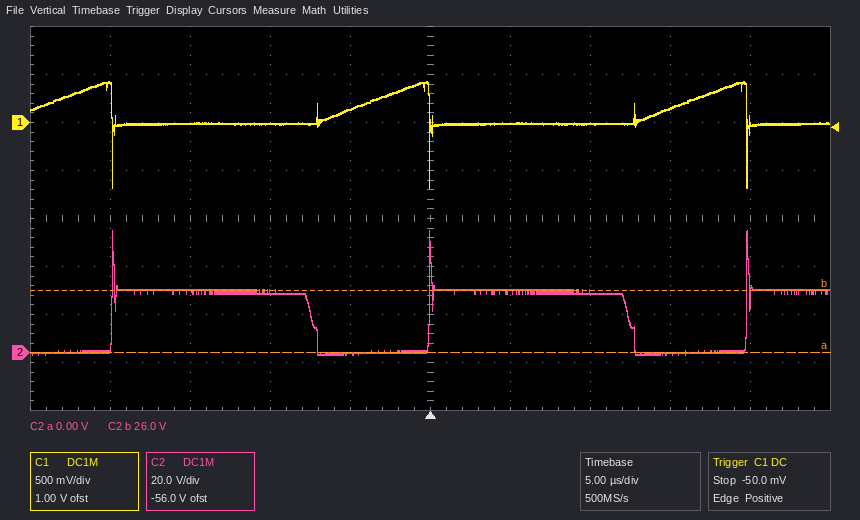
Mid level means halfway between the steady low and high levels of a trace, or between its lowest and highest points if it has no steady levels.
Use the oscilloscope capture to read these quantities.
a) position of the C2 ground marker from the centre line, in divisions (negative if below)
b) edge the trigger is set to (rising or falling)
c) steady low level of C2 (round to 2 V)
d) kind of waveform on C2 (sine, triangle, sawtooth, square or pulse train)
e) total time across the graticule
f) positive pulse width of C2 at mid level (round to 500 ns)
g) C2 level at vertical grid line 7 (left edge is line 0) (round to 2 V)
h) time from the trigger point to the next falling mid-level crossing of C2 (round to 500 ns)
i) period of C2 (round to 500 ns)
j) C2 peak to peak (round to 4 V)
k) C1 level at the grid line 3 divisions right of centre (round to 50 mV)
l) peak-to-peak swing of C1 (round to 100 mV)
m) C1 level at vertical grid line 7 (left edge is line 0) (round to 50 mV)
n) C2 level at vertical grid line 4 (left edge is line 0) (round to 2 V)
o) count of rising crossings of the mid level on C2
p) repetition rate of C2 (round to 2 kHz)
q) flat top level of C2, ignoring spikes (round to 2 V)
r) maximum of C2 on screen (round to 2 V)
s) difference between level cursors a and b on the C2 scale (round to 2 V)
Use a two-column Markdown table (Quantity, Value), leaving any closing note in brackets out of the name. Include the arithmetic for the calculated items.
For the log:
| Quantity | Value |
|---|---|
| position of the C2 ground marker from the centre line, in divisions | -2.8 div |
| edge the trigger is set to | rising |
| steady low level of C2 | 0 V |
| kind of waveform on C2 | pulse train |
| total time across the graticule | 50 µs |
| positive pulse width of C2 at mid level | 12.5 µs |
| C2 level at vertical grid line 7 (left edge is line 0) | 26 V |
| time from the trigger point to the next falling mid-level crossing of C2 | 12.5 µs |
| period of C2 | 20.0 µs |
| C2 peak to peak | 52 V |
| C1 level at the grid line 3 divisions right of centre | 150 mV |
| peak-to-peak swing of C1 | 1.10 V |
| C1 level at vertical grid line 7 (left edge is line 0) | 0 mV |
| C2 level at vertical grid line 4 (left edge is line 0) | 0 V |
| count of rising crossings of the mid level on C2 | 3 |
| repetition rate of C2 | 1 / 20.0 µs ≈ 50 kHz |
| flat top level of C2, ignoring spikes | 26 V |
| maximum of C2 on screen | 52 V |
| difference between level cursors a and b on the C2 scale | 26 V |
